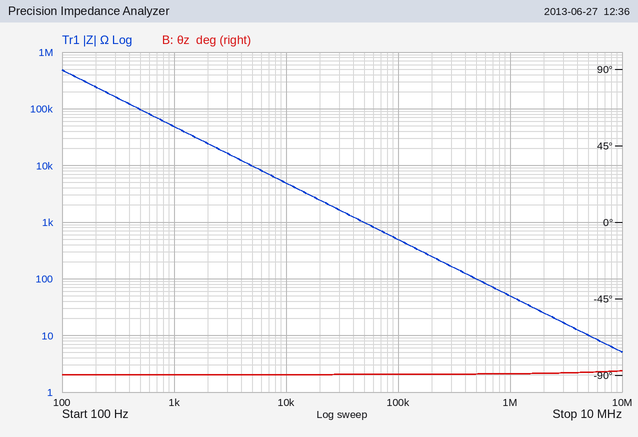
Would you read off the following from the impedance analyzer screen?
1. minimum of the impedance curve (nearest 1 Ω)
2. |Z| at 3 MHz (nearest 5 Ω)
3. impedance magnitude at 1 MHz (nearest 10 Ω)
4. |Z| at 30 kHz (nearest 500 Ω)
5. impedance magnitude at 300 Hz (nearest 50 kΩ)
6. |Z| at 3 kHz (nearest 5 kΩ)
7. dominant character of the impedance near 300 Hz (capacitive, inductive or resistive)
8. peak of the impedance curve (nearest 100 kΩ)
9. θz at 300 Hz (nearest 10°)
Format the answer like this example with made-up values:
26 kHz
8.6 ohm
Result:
5 Ω
15 Ω
50 Ω
1.5 kΩ
150 kΩ
15 kΩ
capacitive
500 kΩ
-90°
